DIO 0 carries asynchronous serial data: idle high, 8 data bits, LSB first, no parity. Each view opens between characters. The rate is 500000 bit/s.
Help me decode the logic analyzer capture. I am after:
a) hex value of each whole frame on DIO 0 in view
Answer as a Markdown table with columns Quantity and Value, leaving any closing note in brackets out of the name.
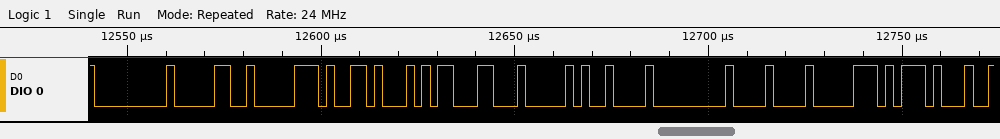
| Quantity | Value |
|---|---|
| hex value of each whole frame on DIO 0 in view | 00, 30, 70, 16, 8D, 04, 09, 00, 08, 70, 17 |
